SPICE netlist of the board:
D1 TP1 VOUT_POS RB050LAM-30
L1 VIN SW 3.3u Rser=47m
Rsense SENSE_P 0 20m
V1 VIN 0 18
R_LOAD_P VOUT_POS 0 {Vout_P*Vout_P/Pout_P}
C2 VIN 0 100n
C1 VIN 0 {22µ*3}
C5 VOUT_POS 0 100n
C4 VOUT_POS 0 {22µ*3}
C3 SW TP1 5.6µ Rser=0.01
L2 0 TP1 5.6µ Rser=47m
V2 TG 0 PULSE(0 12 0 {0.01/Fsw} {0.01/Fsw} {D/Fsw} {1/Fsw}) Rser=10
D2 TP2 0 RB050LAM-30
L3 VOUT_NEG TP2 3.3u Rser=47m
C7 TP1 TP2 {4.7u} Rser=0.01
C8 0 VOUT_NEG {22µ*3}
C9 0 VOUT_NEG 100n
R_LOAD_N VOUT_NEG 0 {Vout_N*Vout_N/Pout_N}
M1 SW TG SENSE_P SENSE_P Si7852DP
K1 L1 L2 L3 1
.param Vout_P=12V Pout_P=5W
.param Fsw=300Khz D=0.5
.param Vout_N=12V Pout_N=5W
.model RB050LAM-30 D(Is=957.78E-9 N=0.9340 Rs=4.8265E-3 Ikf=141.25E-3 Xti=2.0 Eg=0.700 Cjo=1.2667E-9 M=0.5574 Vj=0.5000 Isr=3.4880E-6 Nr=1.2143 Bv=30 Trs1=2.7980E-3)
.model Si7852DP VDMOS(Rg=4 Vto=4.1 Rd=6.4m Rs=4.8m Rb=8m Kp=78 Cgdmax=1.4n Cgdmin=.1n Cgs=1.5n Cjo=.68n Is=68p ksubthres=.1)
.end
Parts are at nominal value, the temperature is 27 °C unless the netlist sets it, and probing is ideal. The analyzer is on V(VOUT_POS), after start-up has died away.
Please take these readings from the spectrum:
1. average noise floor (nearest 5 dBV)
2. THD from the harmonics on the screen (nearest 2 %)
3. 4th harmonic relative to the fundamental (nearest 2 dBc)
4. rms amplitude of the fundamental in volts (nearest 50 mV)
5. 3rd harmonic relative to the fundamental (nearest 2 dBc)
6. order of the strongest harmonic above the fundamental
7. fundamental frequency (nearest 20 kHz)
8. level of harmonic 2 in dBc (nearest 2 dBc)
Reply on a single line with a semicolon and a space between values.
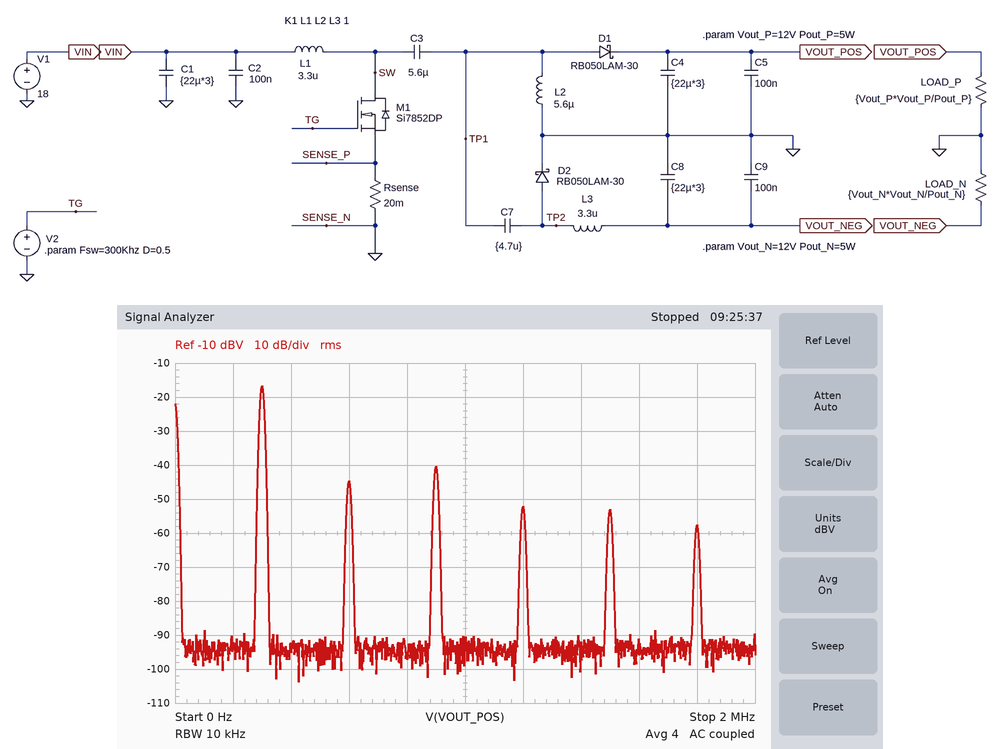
-95 dBV; 8 %; -36 dBc; 150 mV; -24 dBc; 3; 300 kHz; -28 dBc
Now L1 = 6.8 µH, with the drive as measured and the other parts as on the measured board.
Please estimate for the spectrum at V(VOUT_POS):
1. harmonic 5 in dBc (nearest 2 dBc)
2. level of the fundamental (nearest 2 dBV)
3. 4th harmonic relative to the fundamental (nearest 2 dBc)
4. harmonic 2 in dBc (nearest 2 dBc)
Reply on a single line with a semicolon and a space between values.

-22 dBc; -24 dBV; -20 dBc; -8 dBc
